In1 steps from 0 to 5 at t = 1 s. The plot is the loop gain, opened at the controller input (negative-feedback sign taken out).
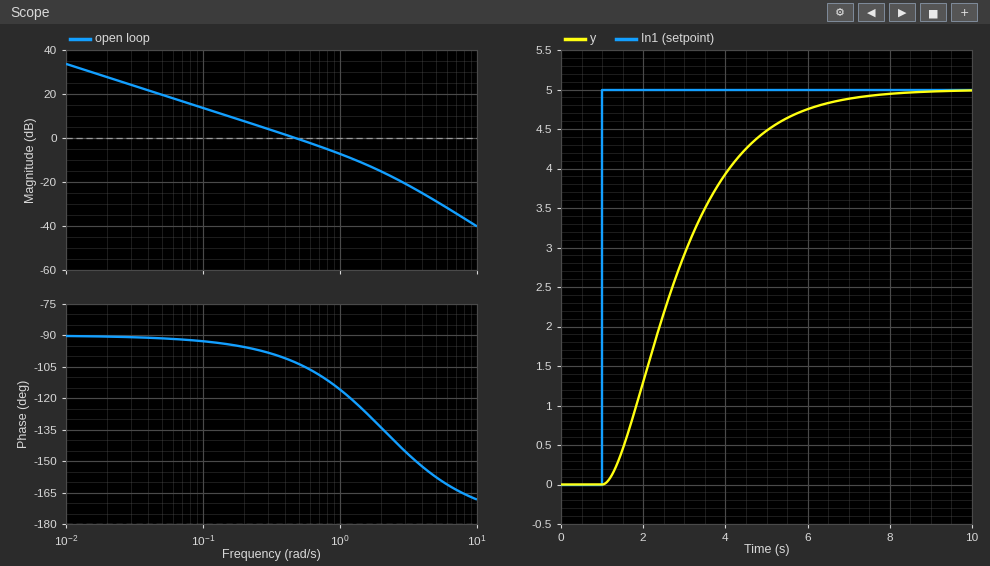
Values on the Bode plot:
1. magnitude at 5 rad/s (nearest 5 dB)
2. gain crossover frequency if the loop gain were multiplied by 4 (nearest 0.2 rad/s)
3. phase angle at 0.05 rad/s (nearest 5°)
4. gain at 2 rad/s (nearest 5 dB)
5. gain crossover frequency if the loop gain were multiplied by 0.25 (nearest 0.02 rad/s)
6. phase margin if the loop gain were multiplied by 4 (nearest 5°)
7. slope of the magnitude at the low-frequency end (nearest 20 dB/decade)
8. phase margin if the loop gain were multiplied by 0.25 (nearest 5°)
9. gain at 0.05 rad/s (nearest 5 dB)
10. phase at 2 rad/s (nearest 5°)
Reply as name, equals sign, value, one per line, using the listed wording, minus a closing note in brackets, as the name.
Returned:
magnitude at 5 rad/s = -30 dB
gain crossover frequency if the loop gain were multiplied by 4 = 1.6 rad/s
phase angle at 0.05 rad/s = -90°
gain at 2 rad/s = -15 dB
gain crossover frequency if the loop gain were multiplied by 0.25 = 0.12 rad/s
phase margin if the loop gain were multiplied by 4 = 55°
slope of the magnitude at the low-frequency end = -20 dB/decade
phase margin if the loop gain were multiplied by 0.25 = 85°
gain at 0.05 rad/s = 20 dB
phase at 2 rad/s = -135°
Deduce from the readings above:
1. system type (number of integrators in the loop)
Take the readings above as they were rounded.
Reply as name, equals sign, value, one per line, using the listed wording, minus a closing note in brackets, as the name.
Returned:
system type = 1
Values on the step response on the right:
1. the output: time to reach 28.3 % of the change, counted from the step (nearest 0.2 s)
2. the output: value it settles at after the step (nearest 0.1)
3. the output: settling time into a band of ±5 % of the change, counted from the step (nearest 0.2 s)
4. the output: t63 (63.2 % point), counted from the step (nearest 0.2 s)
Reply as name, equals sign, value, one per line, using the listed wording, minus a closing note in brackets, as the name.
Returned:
the output: time to reach 28.3 % of the change, counted from the step = 1.0 s
the output: value it settles at after the step = 5.0
the output: settling time into a band of ±5 % of the change, counted from the step = 5.0 s
the output: t63 (63.2 % point), counted from the step = 2.2 s
